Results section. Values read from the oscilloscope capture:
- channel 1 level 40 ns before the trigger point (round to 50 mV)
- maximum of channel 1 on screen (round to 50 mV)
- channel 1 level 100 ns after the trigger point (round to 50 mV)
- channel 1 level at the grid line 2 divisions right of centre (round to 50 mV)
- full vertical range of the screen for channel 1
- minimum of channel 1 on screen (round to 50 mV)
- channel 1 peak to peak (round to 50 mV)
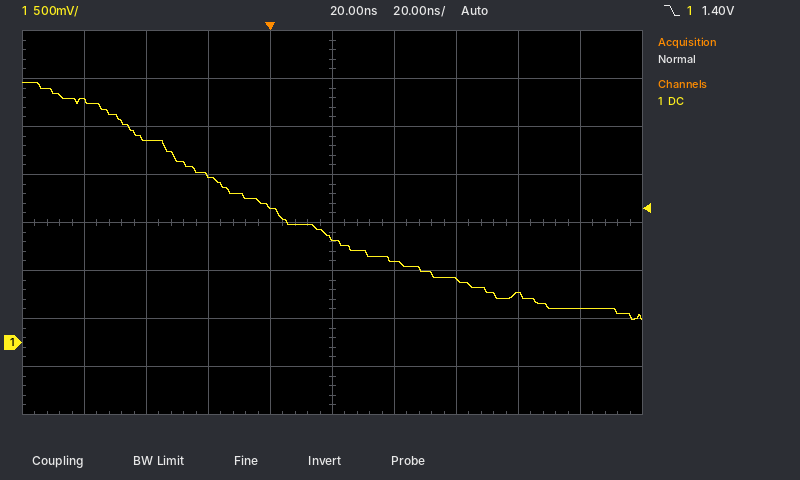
2.10 V
2.70 V
350 mV
650 mV
4 V
250 mV
2.45 V
